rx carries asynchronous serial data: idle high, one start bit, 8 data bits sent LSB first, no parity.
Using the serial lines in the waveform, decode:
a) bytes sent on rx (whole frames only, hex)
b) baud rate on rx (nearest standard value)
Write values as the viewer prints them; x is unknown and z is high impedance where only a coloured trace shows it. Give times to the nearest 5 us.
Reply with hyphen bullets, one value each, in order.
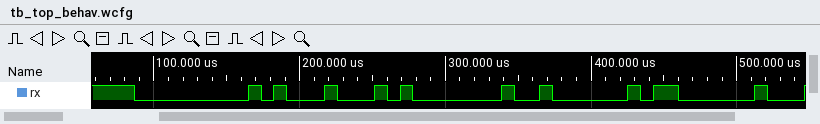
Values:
- 00, 11, 01, 02, 03
- 115200 baud
